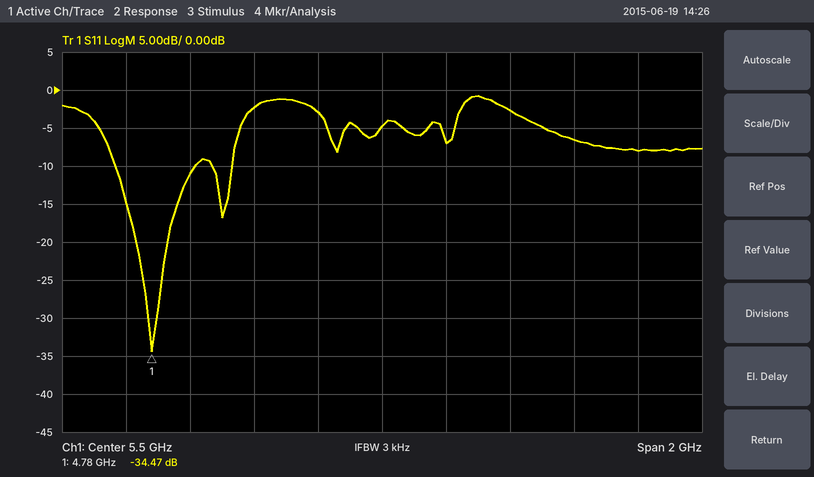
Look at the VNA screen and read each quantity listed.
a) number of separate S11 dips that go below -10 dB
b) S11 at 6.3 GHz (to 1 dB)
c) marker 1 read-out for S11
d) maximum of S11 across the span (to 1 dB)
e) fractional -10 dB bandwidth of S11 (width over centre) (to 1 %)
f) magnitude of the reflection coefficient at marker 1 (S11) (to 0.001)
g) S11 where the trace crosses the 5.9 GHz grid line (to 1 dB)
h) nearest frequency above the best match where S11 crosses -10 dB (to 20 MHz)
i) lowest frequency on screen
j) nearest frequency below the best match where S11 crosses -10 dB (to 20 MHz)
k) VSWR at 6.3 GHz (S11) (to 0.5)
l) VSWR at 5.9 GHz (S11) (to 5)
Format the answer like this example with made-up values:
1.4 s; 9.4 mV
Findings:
2; -8 dB; -34.47 dB; -1 dB; 5 %; 0.019; -3 dB; 4.92 GHz; 4.5 GHz; 4.66 GHz; 2.5; 5
